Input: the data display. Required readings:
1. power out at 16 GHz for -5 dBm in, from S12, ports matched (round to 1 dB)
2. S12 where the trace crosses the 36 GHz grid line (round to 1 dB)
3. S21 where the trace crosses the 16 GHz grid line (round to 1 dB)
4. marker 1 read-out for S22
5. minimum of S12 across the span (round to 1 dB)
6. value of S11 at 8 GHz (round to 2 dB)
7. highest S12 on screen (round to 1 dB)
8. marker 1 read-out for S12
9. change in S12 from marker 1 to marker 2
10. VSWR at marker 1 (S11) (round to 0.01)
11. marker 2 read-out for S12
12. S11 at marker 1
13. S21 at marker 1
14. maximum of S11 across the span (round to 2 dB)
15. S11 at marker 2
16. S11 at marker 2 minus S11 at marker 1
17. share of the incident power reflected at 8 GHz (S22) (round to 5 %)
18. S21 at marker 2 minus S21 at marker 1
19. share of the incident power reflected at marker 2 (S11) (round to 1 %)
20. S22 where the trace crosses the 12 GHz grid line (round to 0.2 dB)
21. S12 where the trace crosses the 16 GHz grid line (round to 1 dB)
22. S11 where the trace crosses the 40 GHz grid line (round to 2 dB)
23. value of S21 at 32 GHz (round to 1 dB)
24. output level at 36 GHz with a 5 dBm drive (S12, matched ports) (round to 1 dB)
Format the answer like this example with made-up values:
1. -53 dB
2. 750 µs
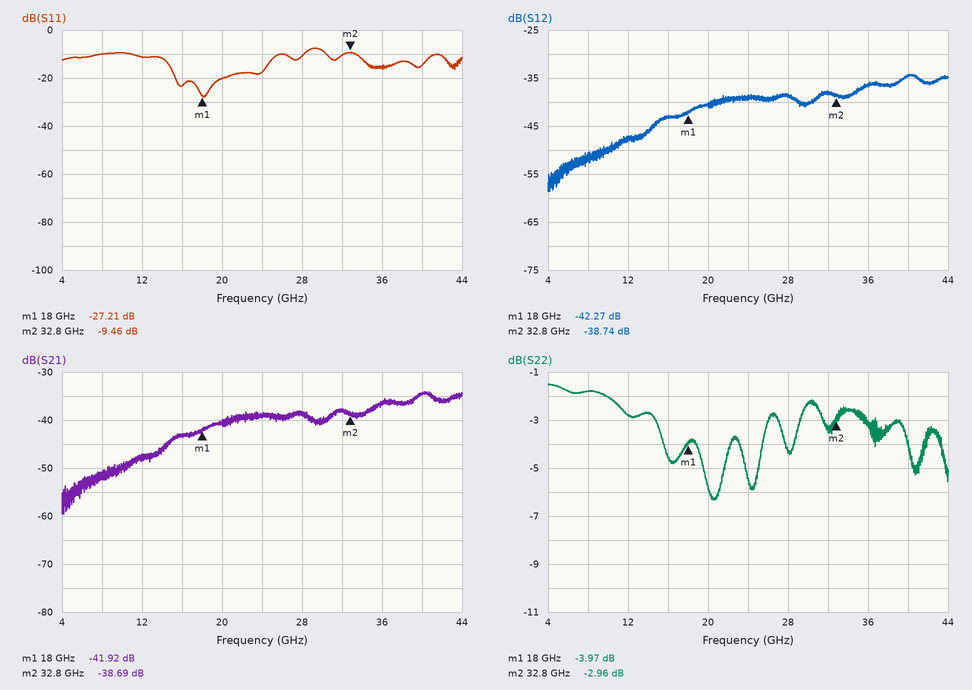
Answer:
1. -48 dBm
2. -36 dB
3. -43 dB
4. -3.97 dB
5. -59 dB
6. -10 dB
7. -34 dB
8. -42.27 dB
9. 3.53 dB
10. 1.09
11. -38.74 dB
12. -27.21 dB
13. -41.92 dB
14. -8 dB
15. -9.46 dB
16. 17.75 dB
17. 65 %
18. 3.23 dB
19. 11 %
20. -2.8 dB
21. -43 dB
22. -14 dB
23. -38 dB
24. -31 dBm
